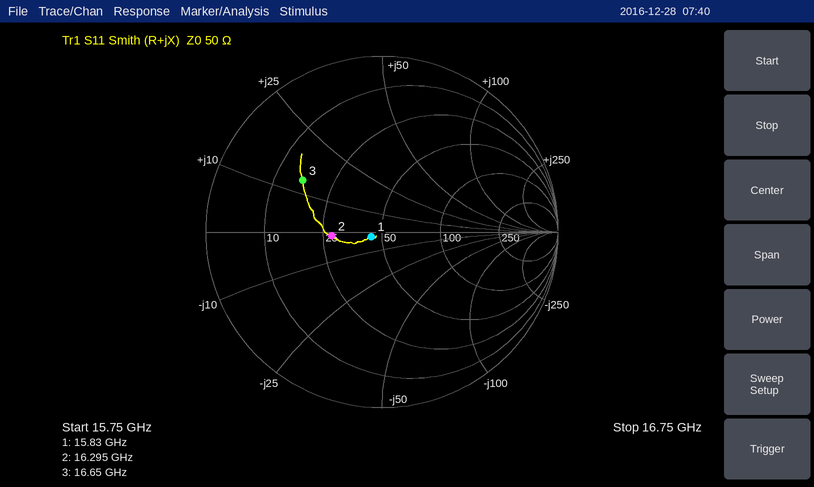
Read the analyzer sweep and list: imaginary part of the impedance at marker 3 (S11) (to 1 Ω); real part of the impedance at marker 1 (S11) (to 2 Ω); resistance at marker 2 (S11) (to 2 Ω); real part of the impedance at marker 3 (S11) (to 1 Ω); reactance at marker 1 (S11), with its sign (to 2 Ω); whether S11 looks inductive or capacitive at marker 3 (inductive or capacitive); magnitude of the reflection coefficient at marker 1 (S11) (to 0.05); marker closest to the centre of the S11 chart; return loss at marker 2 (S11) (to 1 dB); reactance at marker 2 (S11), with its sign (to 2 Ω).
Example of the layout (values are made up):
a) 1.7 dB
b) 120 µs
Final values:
a) +13 Ω
b) 44 Ω
c) 28 Ω
d) 16 Ω
e) -2 Ω
f) inductive
g) 0.05
h) marker 1
i) 11 dB
j) -2 Ω
